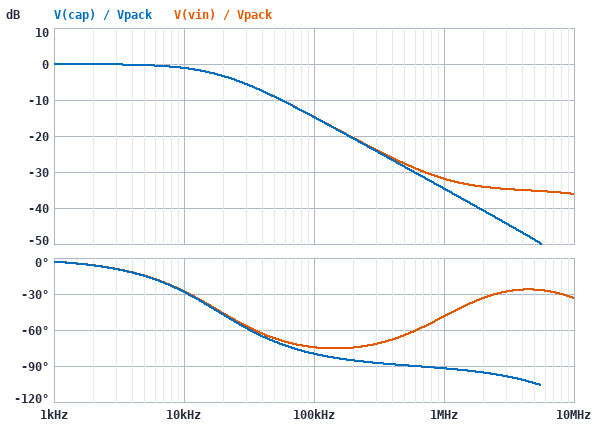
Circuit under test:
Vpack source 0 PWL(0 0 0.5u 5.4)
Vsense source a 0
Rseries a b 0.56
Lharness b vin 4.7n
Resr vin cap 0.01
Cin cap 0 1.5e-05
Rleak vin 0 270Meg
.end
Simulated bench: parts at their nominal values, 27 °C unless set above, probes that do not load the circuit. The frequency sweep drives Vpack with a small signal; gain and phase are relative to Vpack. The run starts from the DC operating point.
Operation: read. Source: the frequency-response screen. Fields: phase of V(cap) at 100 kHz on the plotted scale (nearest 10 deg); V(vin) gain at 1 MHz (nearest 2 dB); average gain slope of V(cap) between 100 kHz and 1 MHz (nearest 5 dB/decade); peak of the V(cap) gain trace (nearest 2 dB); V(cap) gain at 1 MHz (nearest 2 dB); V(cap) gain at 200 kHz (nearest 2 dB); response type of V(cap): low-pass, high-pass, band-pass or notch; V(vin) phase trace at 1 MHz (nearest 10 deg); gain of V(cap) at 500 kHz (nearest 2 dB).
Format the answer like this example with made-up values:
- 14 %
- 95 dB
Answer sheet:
- -80 deg
- -32 dB
- -20 dB/decade
- 0 dB
- -34 dB
- -20 dB
- low-pass
- -50 deg
- -28 dB
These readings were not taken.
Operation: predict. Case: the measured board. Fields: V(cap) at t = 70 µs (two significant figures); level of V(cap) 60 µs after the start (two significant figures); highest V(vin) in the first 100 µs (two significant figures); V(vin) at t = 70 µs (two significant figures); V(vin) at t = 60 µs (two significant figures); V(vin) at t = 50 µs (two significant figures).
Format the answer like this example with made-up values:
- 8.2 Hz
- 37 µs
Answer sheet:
- 5.4 V
- 5.4 V
- 5.4 V
- 5.4 V
- 5.4 V
- 5.4 V
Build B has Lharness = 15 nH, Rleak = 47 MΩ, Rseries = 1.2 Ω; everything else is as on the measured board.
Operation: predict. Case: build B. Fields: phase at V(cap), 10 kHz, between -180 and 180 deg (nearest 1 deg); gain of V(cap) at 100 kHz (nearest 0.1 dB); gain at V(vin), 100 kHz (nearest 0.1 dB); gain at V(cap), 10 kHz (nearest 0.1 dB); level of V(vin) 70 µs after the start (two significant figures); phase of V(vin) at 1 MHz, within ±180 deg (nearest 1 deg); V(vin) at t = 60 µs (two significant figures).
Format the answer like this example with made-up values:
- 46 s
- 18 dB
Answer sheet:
- -49 deg
- -21.2 dB
- -21.1 dB
- -3.6 dB
- 5.3 V
- -51 deg
- 5.2 V
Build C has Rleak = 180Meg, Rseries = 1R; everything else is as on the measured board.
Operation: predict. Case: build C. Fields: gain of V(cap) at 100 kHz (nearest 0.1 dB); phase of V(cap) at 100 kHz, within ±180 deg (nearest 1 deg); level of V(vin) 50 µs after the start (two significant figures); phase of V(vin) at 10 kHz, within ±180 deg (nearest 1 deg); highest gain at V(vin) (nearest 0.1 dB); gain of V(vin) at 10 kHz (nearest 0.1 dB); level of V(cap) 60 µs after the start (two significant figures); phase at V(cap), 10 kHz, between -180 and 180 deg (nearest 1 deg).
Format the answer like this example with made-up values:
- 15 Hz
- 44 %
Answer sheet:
- -19.6 dB
- -84 deg
- 5.2 V
- -43 deg
- 0 dB
- -2.8 dB
- 5.3 V
- -44 deg
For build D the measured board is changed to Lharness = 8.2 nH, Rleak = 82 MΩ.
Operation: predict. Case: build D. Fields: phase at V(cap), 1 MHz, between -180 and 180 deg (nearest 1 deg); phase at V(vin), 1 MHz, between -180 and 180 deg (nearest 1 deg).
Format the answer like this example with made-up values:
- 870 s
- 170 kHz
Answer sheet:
- -94 deg
- -51 deg
